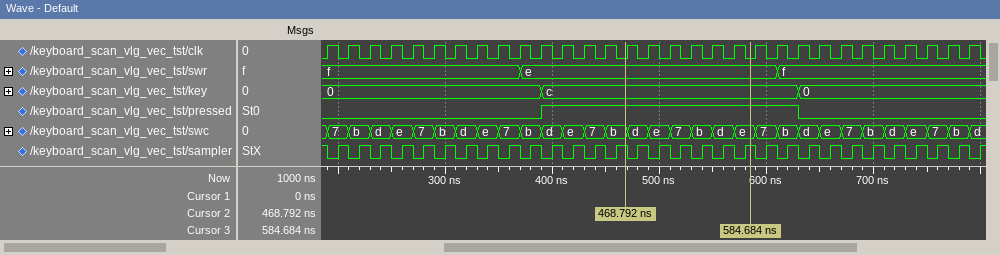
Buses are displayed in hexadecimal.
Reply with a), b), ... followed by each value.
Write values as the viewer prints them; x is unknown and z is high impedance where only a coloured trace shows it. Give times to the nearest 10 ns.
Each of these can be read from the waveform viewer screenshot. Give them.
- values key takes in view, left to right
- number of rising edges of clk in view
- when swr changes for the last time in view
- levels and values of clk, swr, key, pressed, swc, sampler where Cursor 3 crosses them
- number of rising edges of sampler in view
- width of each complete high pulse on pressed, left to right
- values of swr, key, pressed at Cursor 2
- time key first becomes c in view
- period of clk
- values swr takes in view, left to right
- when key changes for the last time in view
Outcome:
a) 0, c, 0
b) 31
c) 610 ns
d) clk=0, swr=e, key=c, pressed=1, swc=e, sampler=1
e) 31
f) 240 ns
g) swr=e, key=c, pressed=1
h) 390 ns
i) 20 ns
j) f, e, f
k) 630 ns
